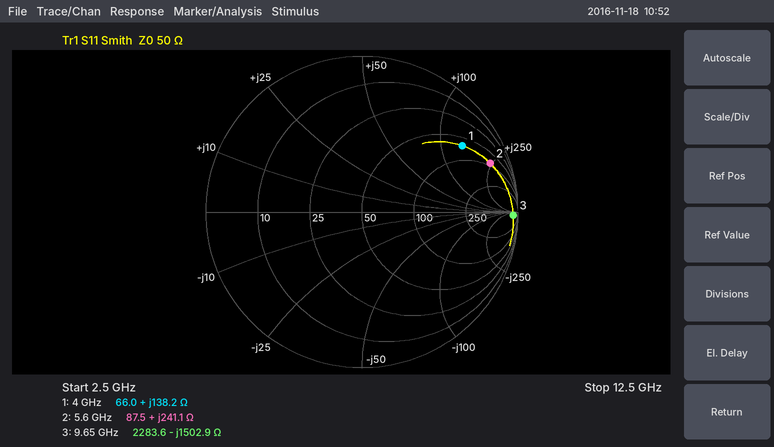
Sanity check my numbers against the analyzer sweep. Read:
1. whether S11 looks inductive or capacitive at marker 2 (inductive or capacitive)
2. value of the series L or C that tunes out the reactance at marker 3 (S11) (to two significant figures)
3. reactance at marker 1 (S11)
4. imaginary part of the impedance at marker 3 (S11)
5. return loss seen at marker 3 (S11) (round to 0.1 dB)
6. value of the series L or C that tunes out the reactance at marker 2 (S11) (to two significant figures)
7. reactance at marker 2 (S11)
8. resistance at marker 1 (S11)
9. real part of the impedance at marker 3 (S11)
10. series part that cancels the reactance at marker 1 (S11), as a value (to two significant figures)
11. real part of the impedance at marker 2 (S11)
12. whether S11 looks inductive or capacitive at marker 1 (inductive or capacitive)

inductive
25 nH
+138.2 Ω
-1502.9 Ω
0.3 dB
120 fF
+241.1 Ω
66.0 Ω
2283.6 Ω
290 fF
87.5 Ω
inductive
